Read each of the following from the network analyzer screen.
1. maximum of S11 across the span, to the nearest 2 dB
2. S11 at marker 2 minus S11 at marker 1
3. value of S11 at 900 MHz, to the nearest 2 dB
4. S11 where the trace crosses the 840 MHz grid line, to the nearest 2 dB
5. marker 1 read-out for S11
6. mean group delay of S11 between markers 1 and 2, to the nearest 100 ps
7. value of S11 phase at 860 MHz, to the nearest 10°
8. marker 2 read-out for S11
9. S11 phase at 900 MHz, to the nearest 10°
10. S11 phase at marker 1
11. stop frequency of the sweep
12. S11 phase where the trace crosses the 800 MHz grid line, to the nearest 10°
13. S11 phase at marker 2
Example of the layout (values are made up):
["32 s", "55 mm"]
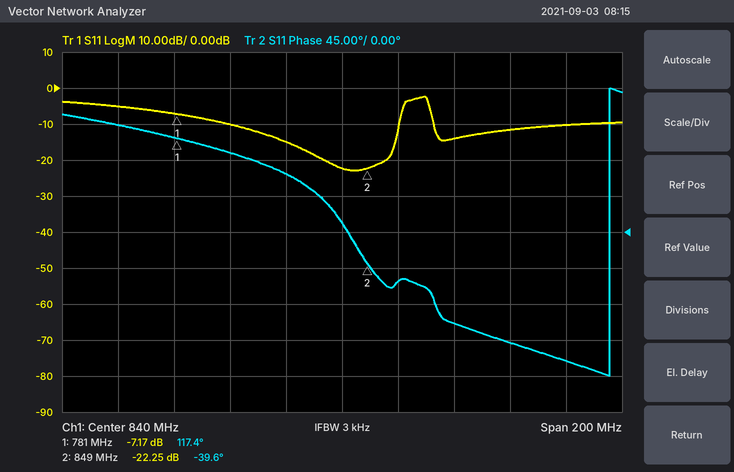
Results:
["-2 dB", "-15.08 dB", "-12 dB", "-22 dB", "-7.17 dB", "6.4 ns", "-60°", "-22.25 dB", "-140°", "117.4°", "940 MHz", "100°", "-39.6°"]
